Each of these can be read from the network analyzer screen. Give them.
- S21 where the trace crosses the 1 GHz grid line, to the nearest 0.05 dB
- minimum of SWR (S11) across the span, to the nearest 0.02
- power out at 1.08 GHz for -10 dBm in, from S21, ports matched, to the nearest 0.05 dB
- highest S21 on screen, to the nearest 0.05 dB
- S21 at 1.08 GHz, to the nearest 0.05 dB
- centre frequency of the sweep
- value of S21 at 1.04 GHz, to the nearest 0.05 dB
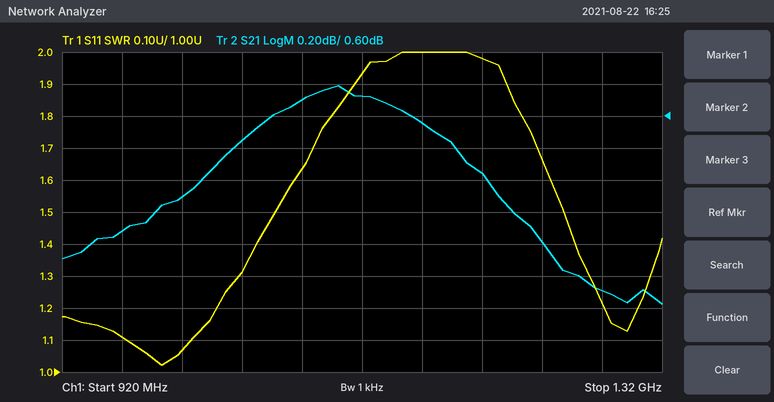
0.10 dB
1.02
-9.30 dBm
0.80 dB
0.70 dB
1.12 GHz
0.45 dB
